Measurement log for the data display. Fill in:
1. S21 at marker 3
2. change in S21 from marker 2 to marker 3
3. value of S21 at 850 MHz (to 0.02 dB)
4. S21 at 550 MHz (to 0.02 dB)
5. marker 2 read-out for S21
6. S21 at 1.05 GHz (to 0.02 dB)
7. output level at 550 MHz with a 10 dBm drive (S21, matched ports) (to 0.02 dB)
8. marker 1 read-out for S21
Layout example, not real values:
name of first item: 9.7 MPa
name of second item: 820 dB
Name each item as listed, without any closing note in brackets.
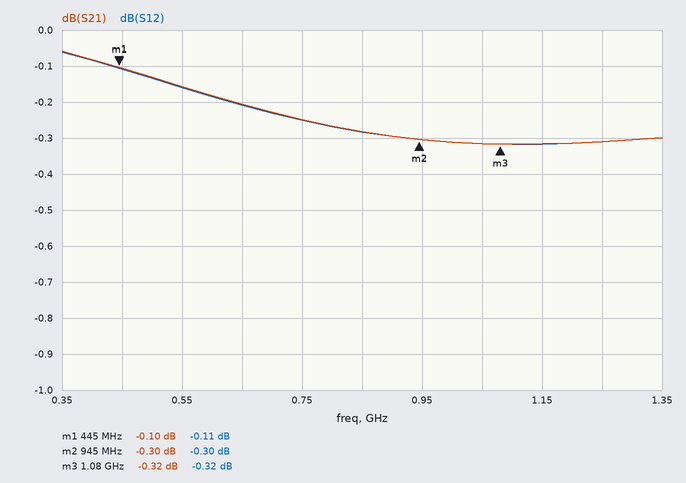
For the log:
S21 at marker 3: -0.32 dB
change in S21 from marker 2 to marker 3: -0.02 dB
value of S21 at 850 MHz: -0.28 dB
S21 at 550 MHz: -0.16 dB
marker 2 read-out for S21: -0.30 dB
S21 at 1.05 GHz: -0.32 dB
output level at 550 MHz with a 10 dBm drive (S21, matched ports): 9.84 dBm
marker 1 read-out for S21: -0.10 dB
